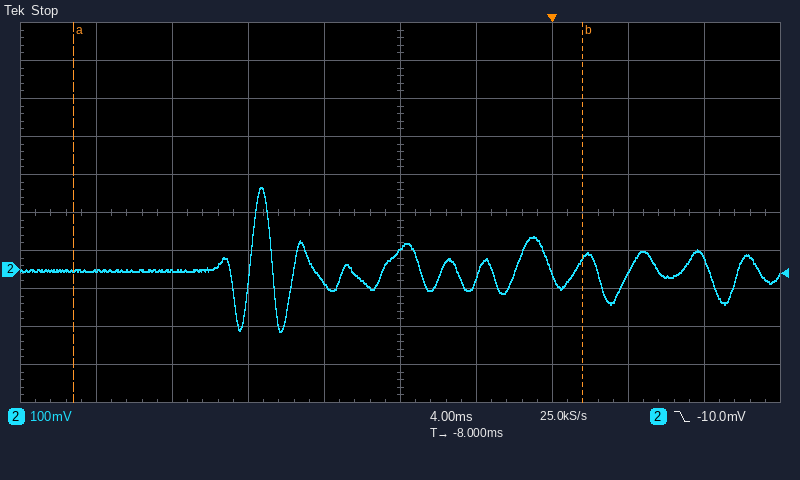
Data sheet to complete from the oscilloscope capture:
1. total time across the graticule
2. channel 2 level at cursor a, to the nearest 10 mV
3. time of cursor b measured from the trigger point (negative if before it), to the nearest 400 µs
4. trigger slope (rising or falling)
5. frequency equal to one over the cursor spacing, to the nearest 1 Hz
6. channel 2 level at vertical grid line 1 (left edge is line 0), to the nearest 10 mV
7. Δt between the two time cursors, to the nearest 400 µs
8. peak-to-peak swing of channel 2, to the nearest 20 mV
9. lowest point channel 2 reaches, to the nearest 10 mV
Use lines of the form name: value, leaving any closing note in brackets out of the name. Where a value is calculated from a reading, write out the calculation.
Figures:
total time across the graticule: 40 ms
channel 2 level at cursor a, to the nearest 10 mV: 0 mV
time of cursor b measured from the trigger point (negative if before it), to the nearest 400 µs: +1.6 ms
trigger slope: falling
frequency equal to one over the cursor spacing, to the nearest 1 Hz: 1 / 26.8 ms ≈ 37 Hz
channel 2 level at vertical grid line 1 (left edge is line 0), to the nearest 10 mV: 0 mV
Δt between the two time cursors, to the nearest 400 µs: 26.8 ms
peak-to-peak swing of channel 2, to the nearest 20 mV: 380 mV
lowest point channel 2 reaches, to the nearest 10 mV: -160 mV
